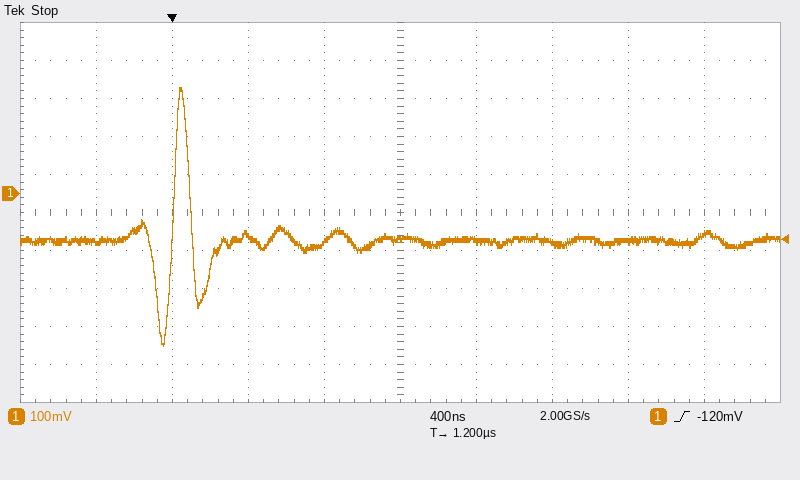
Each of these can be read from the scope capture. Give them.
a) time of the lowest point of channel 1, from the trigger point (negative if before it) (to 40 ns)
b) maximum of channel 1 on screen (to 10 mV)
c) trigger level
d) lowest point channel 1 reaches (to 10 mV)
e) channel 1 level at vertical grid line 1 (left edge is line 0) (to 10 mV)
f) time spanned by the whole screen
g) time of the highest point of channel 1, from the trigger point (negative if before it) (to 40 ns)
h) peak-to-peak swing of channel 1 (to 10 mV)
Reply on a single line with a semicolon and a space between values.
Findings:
-40 ns; 280 mV; -120 mV; -400 mV; -130 mV; 4 µs; +40 ns; 680 mV
